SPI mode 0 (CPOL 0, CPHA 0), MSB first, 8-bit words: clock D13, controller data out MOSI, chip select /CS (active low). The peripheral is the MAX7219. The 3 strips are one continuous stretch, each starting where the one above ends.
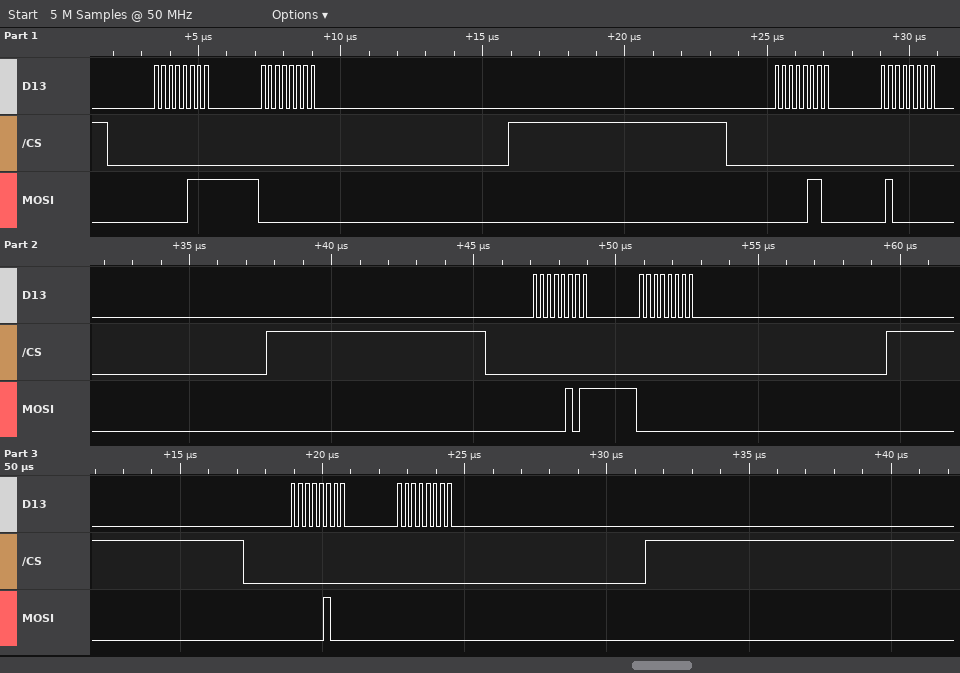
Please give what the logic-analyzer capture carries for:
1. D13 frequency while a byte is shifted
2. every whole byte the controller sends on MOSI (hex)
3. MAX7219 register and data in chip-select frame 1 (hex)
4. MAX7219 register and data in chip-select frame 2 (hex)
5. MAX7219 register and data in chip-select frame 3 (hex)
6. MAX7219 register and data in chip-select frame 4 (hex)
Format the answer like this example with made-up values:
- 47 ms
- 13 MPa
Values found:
- 4 MHz
- 07 00 06 40 05 00 04 00
- register 0x7, data 0x00
- register 0x6, data 0x40
- register 0x5, data 0x00
- register 0x4, data 0x00
